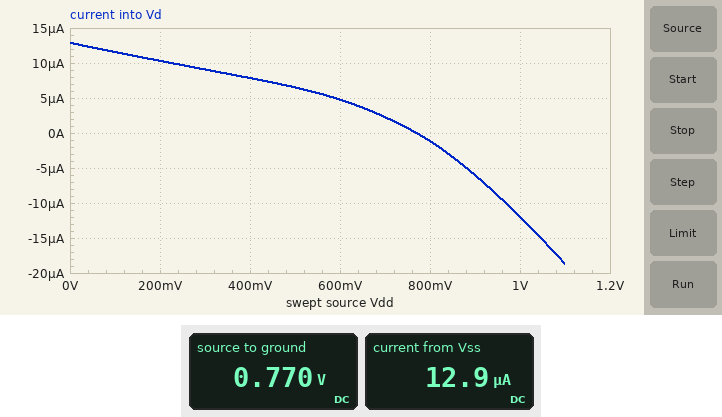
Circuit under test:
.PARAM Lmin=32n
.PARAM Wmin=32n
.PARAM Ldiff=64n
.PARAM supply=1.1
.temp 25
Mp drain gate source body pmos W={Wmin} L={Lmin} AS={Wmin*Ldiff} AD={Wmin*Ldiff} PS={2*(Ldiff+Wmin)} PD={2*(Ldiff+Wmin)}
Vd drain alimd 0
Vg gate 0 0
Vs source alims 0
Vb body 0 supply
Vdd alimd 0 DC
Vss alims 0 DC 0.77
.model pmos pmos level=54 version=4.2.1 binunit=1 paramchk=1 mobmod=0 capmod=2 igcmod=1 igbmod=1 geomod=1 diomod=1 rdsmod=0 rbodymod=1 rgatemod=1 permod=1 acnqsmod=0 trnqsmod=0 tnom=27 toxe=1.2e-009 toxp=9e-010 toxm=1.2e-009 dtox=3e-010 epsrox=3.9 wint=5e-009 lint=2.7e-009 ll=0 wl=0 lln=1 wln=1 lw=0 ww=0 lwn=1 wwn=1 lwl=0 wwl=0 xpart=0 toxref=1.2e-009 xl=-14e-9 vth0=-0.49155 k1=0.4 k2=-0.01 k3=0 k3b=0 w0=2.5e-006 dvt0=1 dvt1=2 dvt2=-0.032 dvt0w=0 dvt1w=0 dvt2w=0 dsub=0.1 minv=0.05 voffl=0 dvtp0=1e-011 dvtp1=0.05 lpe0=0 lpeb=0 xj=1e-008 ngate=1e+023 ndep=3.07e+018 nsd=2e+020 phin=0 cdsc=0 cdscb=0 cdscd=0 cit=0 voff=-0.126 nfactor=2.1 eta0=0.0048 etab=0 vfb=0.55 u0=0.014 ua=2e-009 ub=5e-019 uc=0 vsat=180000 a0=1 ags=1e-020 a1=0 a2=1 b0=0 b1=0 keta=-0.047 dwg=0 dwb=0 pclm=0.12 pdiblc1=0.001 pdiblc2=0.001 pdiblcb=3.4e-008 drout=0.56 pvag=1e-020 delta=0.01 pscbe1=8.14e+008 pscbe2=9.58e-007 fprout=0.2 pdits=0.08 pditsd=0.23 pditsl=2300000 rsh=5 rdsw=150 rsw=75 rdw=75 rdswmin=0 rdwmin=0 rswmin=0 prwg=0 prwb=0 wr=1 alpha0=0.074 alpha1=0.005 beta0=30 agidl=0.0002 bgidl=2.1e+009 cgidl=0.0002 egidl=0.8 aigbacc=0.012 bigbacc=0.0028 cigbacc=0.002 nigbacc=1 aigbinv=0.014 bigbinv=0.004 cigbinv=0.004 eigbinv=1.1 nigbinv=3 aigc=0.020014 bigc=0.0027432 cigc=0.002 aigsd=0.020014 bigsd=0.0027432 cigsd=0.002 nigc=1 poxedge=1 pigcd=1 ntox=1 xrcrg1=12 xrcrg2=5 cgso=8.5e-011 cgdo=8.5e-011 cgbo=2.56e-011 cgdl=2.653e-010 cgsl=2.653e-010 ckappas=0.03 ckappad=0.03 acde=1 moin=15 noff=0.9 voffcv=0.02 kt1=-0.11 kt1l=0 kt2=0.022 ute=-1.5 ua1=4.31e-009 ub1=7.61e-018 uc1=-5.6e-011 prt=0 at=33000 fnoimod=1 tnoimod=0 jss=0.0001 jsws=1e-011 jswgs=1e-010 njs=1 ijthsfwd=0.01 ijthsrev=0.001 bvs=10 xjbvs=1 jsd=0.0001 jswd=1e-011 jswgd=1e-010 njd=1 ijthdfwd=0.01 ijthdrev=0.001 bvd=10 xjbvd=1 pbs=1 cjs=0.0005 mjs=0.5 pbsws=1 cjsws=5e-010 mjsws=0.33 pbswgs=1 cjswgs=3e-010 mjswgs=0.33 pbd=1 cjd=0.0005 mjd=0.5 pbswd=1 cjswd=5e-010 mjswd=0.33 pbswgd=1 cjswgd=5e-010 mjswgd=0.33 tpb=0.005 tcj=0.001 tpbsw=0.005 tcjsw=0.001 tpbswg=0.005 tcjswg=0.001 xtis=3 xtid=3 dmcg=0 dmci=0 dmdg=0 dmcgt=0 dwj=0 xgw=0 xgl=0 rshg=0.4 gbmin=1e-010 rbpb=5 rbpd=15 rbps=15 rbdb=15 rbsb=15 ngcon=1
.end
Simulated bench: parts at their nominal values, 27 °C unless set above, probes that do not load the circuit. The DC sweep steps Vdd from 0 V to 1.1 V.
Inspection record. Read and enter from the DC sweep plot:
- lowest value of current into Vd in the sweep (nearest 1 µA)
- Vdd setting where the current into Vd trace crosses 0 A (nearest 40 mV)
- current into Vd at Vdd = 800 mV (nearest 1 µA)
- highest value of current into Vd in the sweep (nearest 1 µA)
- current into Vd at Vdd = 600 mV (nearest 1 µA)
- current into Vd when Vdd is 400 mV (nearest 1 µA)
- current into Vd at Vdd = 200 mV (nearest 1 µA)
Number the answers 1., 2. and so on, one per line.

1. -19 µA
2. 760 mV
3. -1 µA
4. 13 µA
5. 5 µA
6. 8 µA
7. 10 µA
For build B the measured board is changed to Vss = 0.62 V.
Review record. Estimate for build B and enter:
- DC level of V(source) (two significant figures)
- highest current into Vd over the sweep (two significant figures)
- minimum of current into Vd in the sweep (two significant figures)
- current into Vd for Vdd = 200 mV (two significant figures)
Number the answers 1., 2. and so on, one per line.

1. 620 mV
2. 4.2 µA
3. -24 µA
4. 2.7 µA
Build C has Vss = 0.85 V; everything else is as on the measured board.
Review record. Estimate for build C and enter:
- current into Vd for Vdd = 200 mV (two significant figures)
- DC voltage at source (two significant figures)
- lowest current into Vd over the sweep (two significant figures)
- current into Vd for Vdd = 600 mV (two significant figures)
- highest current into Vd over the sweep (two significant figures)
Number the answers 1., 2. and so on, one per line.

1. 15 µA
2. 850 mV
3. -15 µA
4. 8.8 µA
5. 18 µA
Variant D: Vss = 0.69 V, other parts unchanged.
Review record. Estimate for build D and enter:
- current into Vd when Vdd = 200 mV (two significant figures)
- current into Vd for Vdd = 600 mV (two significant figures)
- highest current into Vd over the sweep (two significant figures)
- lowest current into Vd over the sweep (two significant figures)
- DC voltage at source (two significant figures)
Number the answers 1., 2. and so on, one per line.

1. 5.8 µA
2. 1.7 µA
3. 7.9 µA
4. -22 µA
5. 690 mV
